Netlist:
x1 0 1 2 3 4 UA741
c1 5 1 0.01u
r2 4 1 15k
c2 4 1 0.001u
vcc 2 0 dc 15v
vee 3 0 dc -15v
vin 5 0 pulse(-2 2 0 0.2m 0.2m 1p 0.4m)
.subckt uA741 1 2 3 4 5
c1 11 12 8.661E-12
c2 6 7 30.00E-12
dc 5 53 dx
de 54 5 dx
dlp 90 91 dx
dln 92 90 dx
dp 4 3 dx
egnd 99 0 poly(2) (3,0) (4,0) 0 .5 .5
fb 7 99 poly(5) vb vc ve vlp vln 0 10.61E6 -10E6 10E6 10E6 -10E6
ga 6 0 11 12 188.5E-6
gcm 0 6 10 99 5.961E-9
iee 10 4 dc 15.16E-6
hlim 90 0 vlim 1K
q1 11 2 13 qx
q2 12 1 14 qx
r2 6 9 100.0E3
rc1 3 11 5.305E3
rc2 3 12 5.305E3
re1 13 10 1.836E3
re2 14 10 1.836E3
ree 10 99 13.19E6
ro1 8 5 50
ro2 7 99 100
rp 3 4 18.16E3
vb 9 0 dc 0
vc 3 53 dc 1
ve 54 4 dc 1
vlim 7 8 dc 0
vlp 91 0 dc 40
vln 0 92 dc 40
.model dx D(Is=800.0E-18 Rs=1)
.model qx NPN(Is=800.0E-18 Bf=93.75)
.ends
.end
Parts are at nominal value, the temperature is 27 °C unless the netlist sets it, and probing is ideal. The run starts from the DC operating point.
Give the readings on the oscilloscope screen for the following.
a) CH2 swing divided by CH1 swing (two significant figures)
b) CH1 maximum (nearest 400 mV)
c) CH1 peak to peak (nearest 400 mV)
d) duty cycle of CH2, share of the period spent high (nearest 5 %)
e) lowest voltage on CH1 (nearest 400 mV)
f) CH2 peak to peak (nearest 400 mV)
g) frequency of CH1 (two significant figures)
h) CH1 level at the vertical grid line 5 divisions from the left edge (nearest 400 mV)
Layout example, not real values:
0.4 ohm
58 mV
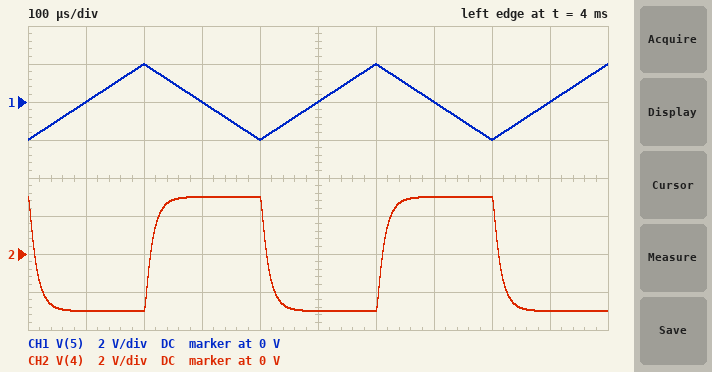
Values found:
1.5
2.0 V
4.0 V
50 %
-2.0 V
6.0 V
2.5 kHz
0 V
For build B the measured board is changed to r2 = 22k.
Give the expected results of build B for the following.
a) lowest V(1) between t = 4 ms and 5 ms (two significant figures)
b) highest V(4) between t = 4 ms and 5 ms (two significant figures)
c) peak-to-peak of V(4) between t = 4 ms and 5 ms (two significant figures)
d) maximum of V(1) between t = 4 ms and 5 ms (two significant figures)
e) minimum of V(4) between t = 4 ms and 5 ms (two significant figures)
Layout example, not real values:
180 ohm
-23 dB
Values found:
-61 mV
4.4 V
8.8 V
61 mV
-4.4 V
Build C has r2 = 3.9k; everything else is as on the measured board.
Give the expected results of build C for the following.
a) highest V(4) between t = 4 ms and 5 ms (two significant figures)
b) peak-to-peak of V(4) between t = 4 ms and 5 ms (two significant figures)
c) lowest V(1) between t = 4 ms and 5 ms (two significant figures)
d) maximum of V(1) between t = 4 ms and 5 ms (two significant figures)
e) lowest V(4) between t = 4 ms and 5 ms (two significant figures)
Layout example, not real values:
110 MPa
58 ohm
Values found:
820 mV
1.6 V
-45 mV
45 mV
-820 mV
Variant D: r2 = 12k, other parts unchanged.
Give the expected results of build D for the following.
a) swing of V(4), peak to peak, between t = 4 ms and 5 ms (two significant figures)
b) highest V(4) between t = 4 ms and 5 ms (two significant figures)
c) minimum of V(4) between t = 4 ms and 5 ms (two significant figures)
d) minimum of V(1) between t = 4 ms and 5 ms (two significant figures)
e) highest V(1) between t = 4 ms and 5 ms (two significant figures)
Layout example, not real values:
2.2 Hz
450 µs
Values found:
4.8 V
2.4 V
-2.4 V
-56 mV
56 mV
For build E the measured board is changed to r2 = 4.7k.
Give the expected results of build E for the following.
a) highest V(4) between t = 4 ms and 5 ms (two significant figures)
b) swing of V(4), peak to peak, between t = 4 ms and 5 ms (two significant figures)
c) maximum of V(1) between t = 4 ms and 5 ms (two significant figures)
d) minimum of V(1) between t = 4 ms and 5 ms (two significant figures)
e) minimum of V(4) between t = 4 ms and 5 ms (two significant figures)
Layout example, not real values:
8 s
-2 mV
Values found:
960 mV
1.9 V
47 mV
-47 mV
-960 mV
